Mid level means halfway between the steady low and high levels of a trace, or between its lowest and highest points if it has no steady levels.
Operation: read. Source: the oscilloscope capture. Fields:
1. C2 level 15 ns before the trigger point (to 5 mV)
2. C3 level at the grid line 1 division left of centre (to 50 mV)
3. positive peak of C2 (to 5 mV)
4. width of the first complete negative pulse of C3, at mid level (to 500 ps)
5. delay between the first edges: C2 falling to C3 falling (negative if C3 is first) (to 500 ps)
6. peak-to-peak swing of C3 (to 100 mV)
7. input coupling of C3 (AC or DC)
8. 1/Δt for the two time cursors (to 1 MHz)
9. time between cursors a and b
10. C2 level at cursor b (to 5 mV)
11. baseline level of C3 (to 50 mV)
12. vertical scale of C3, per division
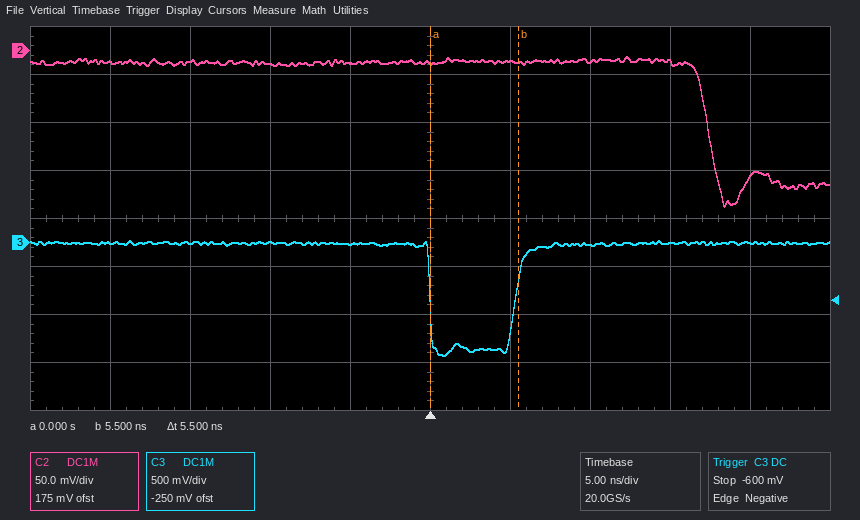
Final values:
-10 mV
0 mV
-5 mV
5.5 ns
-17.5 ns
1.20 V
DC
182 MHz
5.5 ns
-10 mV
0 mV
500 mV
